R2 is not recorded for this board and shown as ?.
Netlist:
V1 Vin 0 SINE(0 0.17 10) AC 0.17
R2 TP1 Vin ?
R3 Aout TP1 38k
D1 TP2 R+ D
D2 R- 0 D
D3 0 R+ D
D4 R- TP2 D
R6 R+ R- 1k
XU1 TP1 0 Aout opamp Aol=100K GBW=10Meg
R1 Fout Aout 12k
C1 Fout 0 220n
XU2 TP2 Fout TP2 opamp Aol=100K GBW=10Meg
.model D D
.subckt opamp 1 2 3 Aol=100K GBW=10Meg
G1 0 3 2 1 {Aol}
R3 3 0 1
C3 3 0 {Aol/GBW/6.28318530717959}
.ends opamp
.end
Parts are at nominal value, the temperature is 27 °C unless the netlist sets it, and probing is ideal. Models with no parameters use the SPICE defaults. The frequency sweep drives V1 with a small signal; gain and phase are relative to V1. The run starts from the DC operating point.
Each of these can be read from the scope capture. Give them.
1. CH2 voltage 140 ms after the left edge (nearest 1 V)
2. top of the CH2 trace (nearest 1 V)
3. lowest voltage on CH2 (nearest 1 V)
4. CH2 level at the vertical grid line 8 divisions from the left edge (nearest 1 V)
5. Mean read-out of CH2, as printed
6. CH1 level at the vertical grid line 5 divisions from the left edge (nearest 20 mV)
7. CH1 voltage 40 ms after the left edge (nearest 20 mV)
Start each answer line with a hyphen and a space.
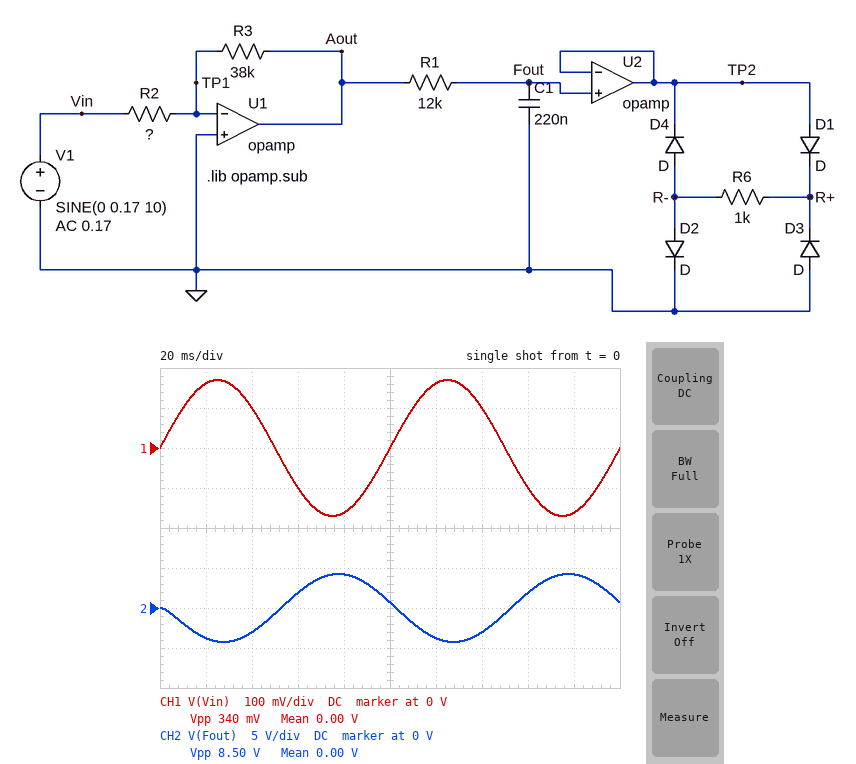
- -3 V
- 4 V
- -4 V
- 2 V
- 0.00 V
- 0 V
- 100 mV
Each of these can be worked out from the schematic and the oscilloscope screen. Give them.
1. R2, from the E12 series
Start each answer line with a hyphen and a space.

- 1.5 kΩ
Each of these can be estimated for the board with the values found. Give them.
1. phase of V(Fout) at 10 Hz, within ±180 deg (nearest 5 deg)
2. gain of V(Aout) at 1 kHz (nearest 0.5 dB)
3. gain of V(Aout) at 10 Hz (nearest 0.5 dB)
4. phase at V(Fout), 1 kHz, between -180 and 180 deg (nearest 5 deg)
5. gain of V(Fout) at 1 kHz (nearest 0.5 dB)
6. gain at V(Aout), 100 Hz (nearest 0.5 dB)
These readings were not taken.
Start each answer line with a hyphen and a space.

- 170 deg
- 28.0 dB
- 28.0 dB
- 95 deg
- 3.5 dB
- 28.0 dB
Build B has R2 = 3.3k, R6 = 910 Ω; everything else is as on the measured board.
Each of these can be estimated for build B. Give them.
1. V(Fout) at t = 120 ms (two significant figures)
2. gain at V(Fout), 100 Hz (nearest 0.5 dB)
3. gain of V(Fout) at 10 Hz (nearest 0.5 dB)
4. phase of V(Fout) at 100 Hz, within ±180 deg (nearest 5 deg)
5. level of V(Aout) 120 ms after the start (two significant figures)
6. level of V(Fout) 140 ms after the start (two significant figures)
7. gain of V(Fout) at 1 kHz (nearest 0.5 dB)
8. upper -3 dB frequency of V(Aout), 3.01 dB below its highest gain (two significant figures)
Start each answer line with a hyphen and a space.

- -1.7 V
- 15.5 dB
- 21.0 dB
- 120 deg
- -1.9 V
- -1.4 V
- -3.0 dB
- 800 kHz
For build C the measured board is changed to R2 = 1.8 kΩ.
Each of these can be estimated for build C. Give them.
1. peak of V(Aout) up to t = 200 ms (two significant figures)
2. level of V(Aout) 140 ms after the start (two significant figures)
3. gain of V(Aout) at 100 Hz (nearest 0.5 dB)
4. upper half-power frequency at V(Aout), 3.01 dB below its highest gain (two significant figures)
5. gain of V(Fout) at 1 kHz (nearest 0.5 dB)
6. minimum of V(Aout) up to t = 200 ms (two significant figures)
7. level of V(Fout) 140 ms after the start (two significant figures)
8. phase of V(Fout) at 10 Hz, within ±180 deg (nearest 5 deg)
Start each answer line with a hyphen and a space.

- 3.6 V
- -2.1 V
- 26.5 dB
- 450 kHz
- 2.0 dB
- -3.6 V
- -2.5 V
- 170 deg
